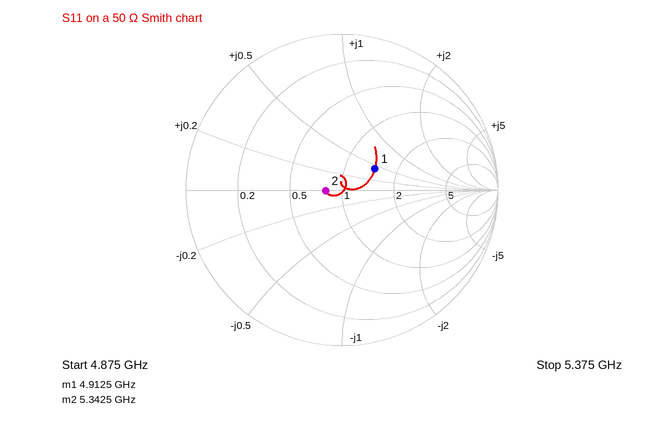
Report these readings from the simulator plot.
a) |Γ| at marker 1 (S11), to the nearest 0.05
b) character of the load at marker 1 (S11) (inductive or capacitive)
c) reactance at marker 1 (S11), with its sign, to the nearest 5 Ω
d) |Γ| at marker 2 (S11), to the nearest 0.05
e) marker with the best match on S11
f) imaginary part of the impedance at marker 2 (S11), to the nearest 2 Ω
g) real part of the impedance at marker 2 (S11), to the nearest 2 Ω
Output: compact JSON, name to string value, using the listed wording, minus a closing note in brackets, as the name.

{"|Γ| at marker 1 (S11), to the nearest 0.05": "0.25", "character of the load at marker 1 (S11)": "inductive", "reactance at marker 1 (S11), with its sign, to the nearest 5 Ω": "+20 Ω", "|Γ| at marker 2 (S11), to the nearest 0.05": "0.10", "marker with the best match on S11": "marker 2", "imaginary part of the impedance at marker 2 (S11), to the nearest 2 Ω": "0 Ω", "real part of the impedance at marker 2 (S11), to the nearest 2 Ω": "40 Ω"}
